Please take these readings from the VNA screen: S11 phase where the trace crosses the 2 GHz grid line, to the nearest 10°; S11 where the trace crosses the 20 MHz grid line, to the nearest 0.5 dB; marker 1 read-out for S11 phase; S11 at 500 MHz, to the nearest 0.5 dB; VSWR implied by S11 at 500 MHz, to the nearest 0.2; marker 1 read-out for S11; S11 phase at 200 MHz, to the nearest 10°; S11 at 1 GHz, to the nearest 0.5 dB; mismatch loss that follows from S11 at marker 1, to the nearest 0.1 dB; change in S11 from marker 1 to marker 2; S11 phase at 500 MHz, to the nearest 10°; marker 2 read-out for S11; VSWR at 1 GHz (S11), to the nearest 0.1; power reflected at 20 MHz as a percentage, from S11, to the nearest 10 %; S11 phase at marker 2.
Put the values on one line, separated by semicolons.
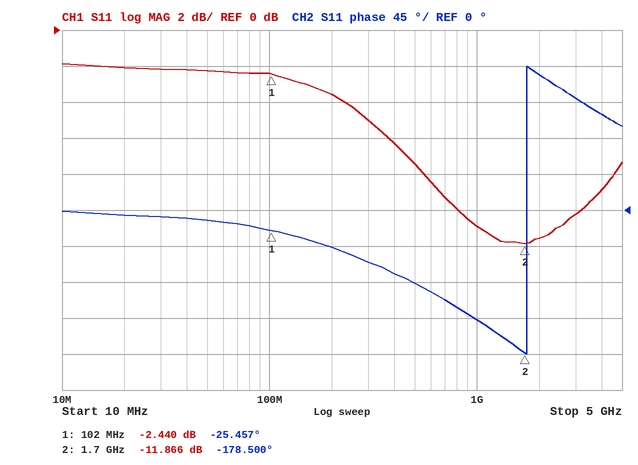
170°; -2.0 dB; -25.457°; -7.5 dB; 2.4; -2.440 dB; -50°; -11.0 dB; 3.7 dB; -9.426 dB; -90°; -11.866 dB; 1.8; 60 %; -178.500°
